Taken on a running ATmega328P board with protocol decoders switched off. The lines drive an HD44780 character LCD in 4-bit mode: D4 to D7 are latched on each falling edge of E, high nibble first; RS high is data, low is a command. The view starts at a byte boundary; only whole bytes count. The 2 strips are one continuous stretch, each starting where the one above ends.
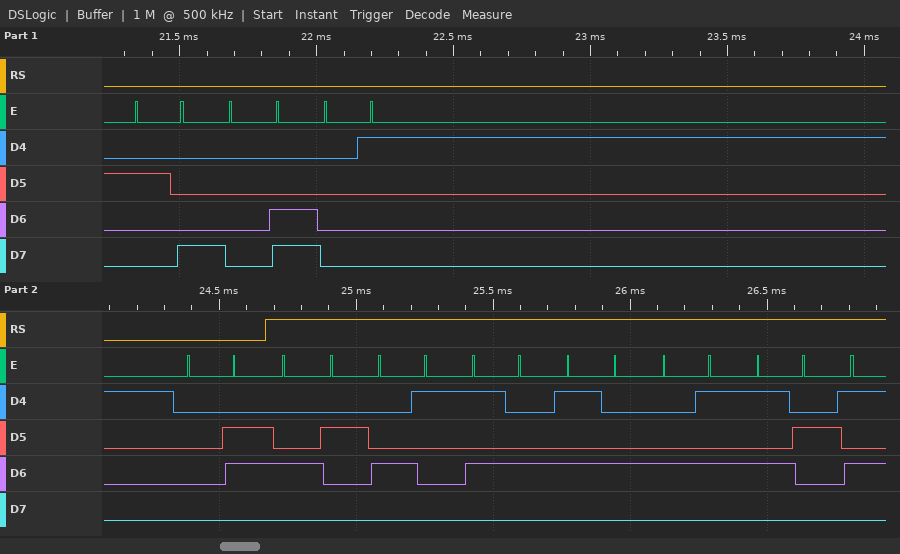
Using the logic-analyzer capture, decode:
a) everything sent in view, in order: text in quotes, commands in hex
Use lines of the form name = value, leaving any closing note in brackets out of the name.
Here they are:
everything sent in view, in order: text in quotes, commands in hex = 0x28 0x0C 0x01 0x06 "BATTER"
